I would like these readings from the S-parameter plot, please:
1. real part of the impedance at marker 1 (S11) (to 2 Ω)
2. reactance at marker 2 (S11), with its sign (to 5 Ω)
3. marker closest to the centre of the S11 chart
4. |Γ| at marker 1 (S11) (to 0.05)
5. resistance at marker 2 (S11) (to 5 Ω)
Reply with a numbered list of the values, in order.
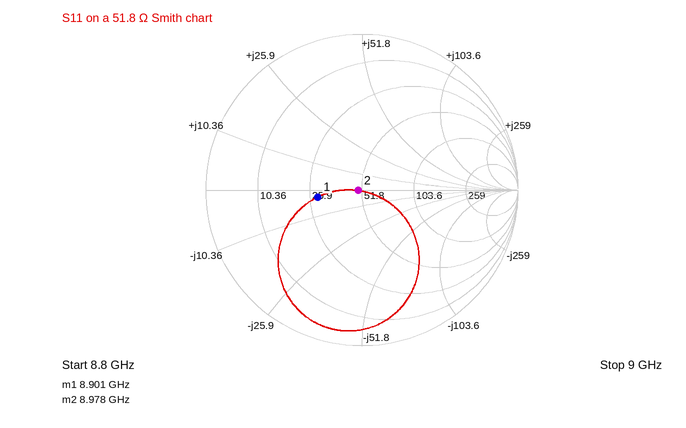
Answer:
1. 28 Ω
2. 0 Ω
3. marker 2
4. 0.30
5. 50 Ω
